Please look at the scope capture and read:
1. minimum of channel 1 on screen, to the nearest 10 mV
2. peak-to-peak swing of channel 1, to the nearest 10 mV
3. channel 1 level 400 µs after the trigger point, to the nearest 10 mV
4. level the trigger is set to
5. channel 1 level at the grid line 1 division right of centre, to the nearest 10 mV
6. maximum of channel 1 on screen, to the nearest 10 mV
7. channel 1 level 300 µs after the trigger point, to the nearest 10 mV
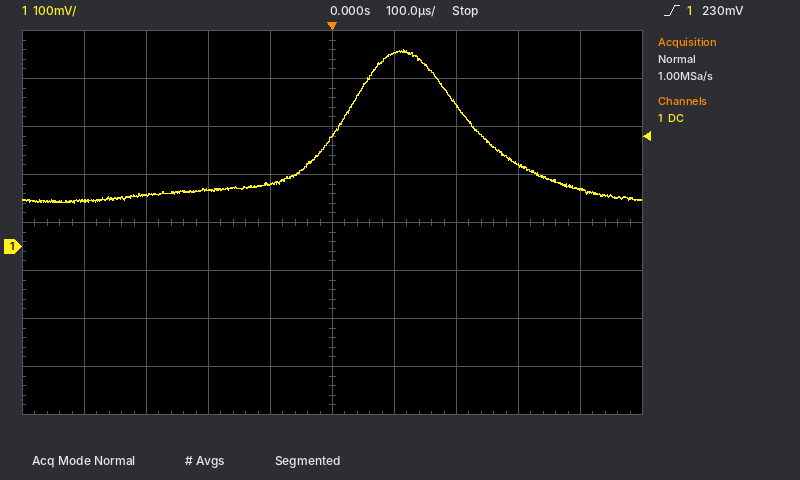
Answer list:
90 mV
320 mV
120 mV
230 mV
400 mV
410 mV
170 mV
